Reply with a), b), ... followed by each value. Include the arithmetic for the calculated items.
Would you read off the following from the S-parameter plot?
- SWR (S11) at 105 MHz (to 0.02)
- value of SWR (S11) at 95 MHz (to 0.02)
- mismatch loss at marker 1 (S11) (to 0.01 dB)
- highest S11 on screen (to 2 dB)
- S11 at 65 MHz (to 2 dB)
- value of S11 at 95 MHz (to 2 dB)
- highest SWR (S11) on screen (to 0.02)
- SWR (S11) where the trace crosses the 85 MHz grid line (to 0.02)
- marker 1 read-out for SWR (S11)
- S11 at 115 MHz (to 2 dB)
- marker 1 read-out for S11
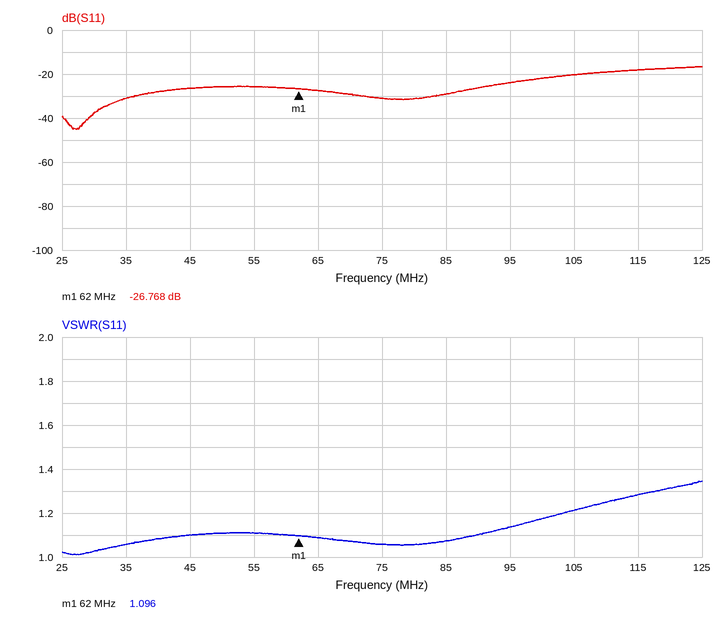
a) 1.22
b) 1.14
c) −10 log10(1 − 10^(-26.768/10)) ≈ 0.01 dB
d) -16 dB
e) -28 dB
f) -24 dB
g) 1.34
h) 1.08
i) 1.096
j) -18 dB
k) -26.768 dB
